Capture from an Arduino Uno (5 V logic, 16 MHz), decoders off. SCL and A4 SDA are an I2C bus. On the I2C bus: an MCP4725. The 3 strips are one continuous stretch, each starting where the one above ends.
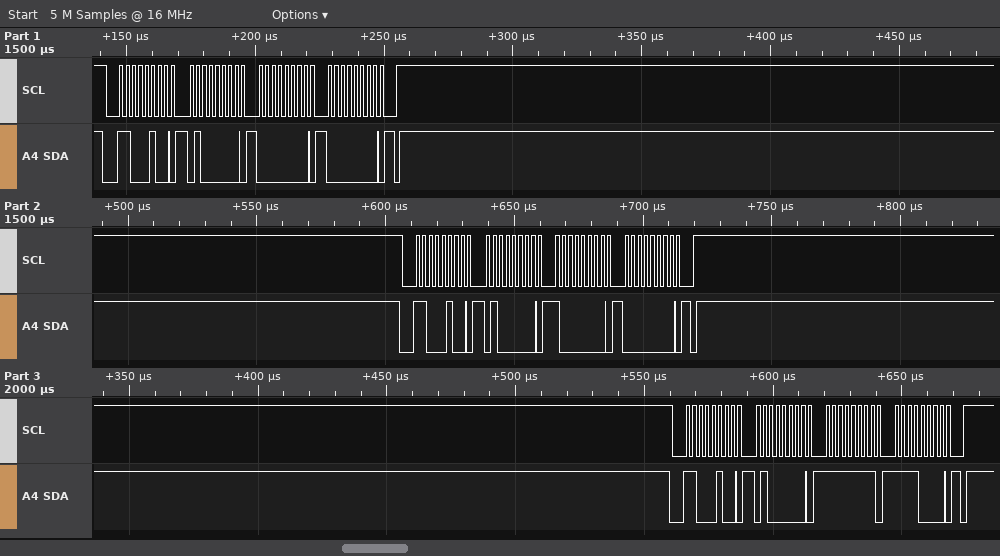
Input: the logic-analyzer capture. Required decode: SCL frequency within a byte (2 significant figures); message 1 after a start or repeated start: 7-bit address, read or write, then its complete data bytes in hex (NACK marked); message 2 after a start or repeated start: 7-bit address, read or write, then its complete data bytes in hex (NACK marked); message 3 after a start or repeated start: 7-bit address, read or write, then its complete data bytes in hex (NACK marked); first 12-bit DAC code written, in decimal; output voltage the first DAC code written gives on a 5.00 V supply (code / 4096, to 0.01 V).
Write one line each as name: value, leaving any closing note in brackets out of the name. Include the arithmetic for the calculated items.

SCL frequency within a byte: 400 kHz
message 1 after a start or repeated start: 7-bit address, read or write, then its complete data bytes in hex: 0x62 write: 40 00 00
message 2 after a start or repeated start: 7-bit address, read or write, then its complete data bytes in hex: 0x62 write: 40 80 00
message 3 after a start or repeated start: 7-bit address, read or write, then its complete data bytes in hex: 0x62 write: 40 FF F0
first 12-bit DAC code written, in decimal: 0
output voltage the first DAC code written gives on a 5.00 V supply: 0 / 4096 x 5.00 V = 0.00 V
